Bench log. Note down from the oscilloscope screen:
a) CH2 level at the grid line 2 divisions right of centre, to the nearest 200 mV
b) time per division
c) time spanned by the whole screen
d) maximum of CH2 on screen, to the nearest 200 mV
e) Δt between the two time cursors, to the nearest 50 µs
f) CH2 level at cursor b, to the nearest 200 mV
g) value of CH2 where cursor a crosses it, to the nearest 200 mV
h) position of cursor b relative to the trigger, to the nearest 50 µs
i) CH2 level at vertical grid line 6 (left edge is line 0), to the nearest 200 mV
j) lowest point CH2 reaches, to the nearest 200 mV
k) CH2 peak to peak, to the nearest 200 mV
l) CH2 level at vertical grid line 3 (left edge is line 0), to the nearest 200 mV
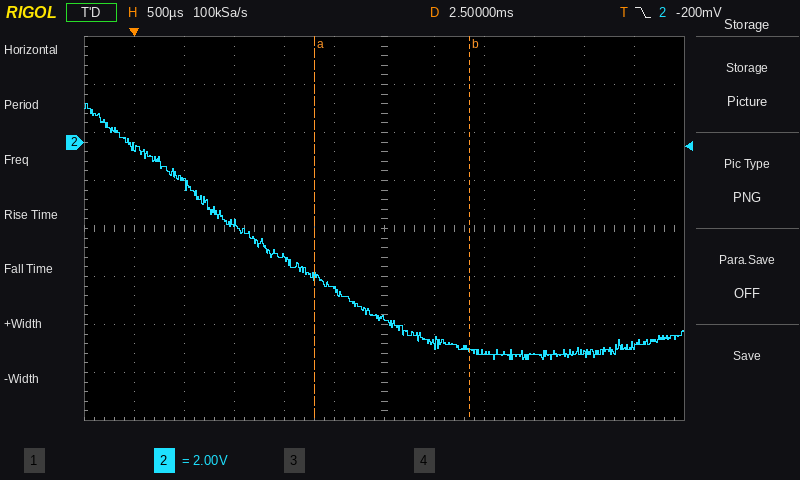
-8.8 V
500 µs
6 ms
1.6 V
1.55 ms
-8.6 V
-5.6 V
+3.35 ms
-7.4 V
-9.0 V
10.6 V
-3.4 V
